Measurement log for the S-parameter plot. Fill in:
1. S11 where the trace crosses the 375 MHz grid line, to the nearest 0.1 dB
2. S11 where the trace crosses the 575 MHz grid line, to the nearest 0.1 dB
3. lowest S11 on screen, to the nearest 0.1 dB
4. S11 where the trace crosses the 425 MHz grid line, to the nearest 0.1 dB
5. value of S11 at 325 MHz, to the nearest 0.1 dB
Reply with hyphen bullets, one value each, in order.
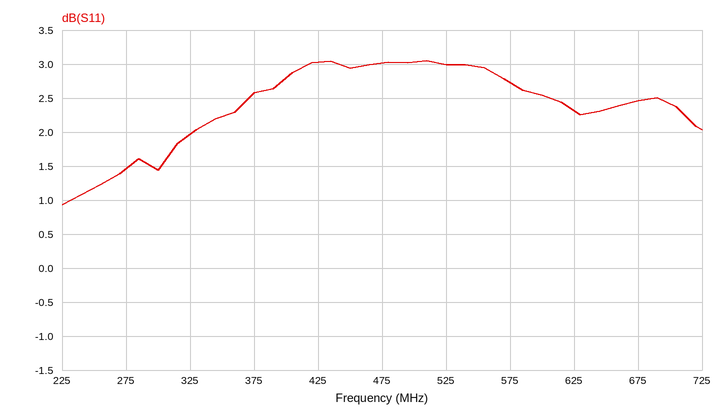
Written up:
- 2.6 dB
- 2.7 dB
- 0.9 dB
- 3.0 dB
- 2.0 dB
